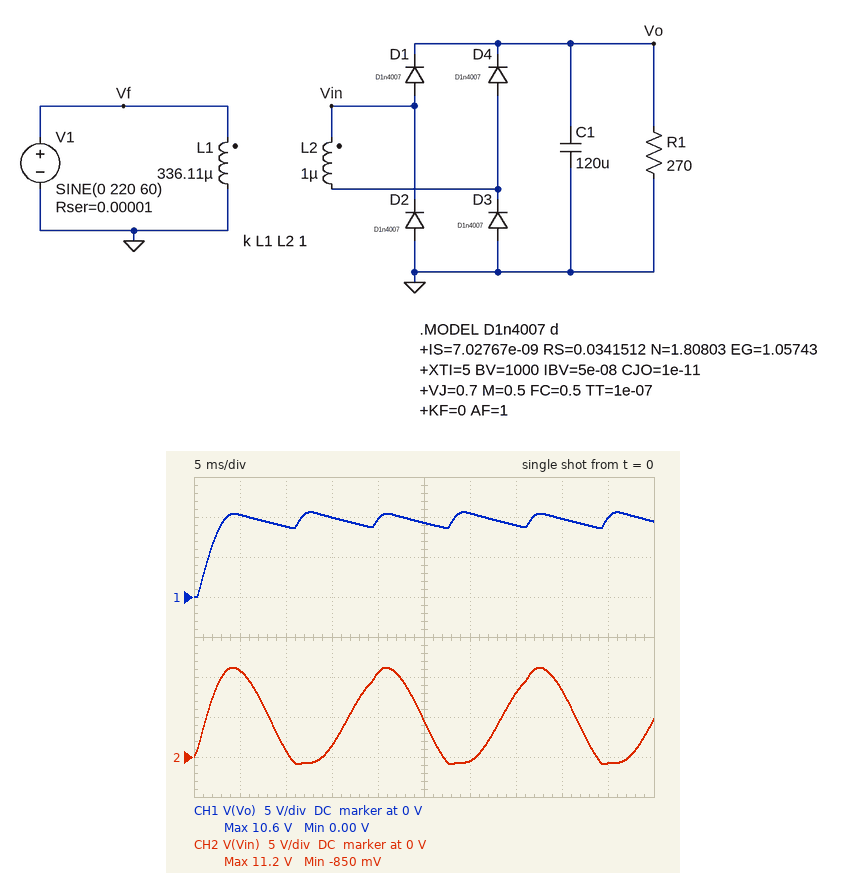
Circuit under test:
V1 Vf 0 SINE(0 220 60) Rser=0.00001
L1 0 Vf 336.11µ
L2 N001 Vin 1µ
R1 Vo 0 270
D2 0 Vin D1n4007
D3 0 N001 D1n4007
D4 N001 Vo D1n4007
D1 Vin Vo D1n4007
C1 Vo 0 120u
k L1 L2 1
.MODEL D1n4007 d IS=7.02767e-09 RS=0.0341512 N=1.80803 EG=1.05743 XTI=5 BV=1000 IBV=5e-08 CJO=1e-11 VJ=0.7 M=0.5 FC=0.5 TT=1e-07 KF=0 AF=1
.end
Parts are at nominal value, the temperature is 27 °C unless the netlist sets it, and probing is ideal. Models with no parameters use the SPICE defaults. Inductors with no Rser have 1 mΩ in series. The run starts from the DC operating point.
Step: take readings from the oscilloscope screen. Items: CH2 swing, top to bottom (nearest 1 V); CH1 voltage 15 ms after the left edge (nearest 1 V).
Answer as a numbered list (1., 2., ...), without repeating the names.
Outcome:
1. 12 V
2. 10 V
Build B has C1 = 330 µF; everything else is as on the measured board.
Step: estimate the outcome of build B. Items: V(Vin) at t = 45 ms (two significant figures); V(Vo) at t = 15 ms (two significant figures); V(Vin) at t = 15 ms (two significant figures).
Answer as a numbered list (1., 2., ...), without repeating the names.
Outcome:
1. -860 mV
2. 10 V
3. 1.6 V
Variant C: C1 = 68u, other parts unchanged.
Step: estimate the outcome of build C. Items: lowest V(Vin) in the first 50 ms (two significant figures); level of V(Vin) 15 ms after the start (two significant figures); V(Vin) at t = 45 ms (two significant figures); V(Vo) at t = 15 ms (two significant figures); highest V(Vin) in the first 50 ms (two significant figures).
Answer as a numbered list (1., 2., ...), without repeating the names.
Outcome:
1. -810 mV
2. 1.2 V
3. -790 mV
4. 9.5 V
5. 11 V
